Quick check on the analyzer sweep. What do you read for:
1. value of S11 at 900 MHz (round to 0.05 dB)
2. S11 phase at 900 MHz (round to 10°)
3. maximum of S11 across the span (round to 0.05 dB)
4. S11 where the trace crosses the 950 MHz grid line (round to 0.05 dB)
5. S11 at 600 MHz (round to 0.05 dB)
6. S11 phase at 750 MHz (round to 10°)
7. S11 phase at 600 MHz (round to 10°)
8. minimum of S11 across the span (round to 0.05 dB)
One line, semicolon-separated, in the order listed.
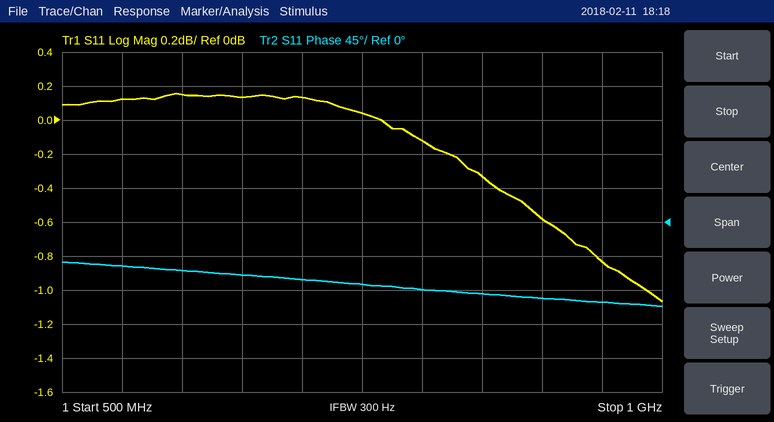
-0.60 dB; -100°; 0.15 dB; -0.85 dB; 0.15 dB; -80°; -60°; -1.05 dB
